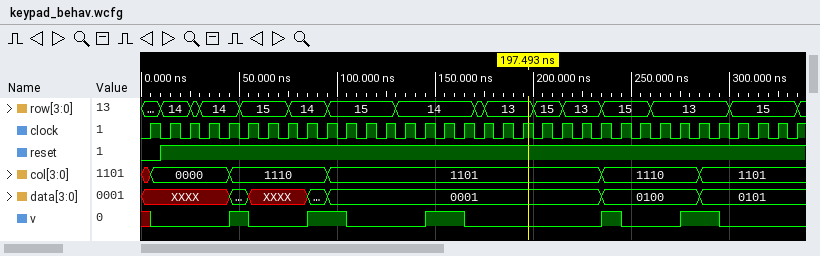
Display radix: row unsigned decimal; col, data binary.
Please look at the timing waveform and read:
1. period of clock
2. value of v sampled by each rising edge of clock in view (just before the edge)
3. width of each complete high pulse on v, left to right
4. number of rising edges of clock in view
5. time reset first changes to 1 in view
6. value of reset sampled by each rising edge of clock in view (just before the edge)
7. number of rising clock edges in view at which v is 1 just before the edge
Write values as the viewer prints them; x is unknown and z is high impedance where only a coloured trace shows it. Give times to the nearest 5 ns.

10 ns
x 0 0 0 0 1 0 0 0 1 1 0 0 0 0 1 1 0 0 0 0 0 0 0 1 0 0 0 1 1 0 0 0 0
10 ns, 20 ns, 20 ns, 10 ns, 20 ns
34
10 ns
0 1 1 1 1 1 1 1 1 1 1 1 1 1 1 1 1 1 1 1 1 1 1 1 1 1 1 1 1 1 1 1 1 1
8
